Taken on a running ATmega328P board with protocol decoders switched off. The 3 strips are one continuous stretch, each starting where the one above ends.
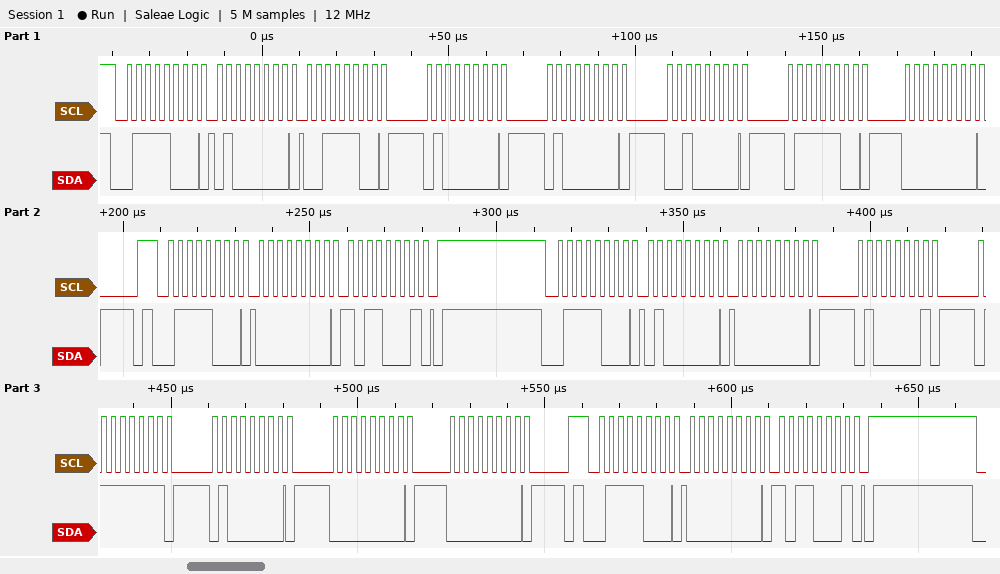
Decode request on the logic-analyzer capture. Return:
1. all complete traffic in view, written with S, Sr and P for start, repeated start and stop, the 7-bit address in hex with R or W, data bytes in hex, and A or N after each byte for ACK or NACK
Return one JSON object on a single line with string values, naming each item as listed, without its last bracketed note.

{"all complete traffic in view, written with S, Sr and P for start, repeated start and stop, the 7-bit address in hex with R or W, data bytes in hex, and A or N after each byte for ACK or NACK": "S 3CW A 40 A 3C A 40 A 40 A 20 A 7C A 00 A P S 3CW A 00 A B1 A P S 3CW A 40 A 00 A 41 A 7F A 40 A 00 A 00 A P S 3CW A 00 A B1 A P"}
